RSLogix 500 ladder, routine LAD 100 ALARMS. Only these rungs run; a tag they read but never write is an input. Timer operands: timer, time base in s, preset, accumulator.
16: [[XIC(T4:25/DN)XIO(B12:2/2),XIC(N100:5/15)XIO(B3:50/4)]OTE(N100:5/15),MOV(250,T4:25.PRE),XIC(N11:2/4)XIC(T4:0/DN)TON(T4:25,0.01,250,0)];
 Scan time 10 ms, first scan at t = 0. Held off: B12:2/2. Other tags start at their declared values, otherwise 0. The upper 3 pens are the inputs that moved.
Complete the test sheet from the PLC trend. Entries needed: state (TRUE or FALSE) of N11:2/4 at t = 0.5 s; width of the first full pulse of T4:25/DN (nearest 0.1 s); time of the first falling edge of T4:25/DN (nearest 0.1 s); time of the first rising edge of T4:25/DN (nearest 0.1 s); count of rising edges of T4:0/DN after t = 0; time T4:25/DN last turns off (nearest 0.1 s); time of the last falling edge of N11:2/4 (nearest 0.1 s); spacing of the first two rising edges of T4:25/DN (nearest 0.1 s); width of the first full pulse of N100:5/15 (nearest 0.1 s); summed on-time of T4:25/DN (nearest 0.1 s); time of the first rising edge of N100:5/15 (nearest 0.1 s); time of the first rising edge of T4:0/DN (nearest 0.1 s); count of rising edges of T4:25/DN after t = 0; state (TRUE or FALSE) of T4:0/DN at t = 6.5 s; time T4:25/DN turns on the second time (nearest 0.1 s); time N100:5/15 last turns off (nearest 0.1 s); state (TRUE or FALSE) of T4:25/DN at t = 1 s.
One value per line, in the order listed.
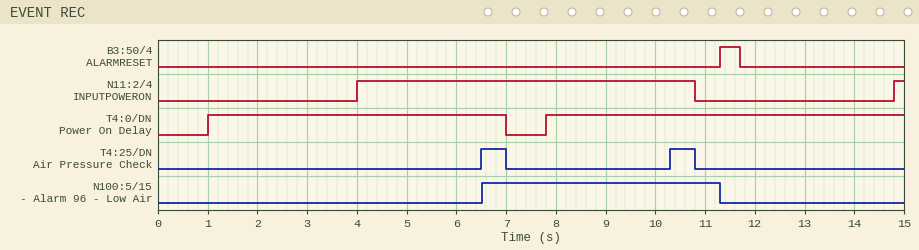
FALSE
0.5 s
7.0 s
6.5 s
2
10.8 s
10.8 s
3.8 s
4.8 s
1.0 s
6.5 s
1.0 s
2
TRUE
10.3 s
11.3 s
FALSE
